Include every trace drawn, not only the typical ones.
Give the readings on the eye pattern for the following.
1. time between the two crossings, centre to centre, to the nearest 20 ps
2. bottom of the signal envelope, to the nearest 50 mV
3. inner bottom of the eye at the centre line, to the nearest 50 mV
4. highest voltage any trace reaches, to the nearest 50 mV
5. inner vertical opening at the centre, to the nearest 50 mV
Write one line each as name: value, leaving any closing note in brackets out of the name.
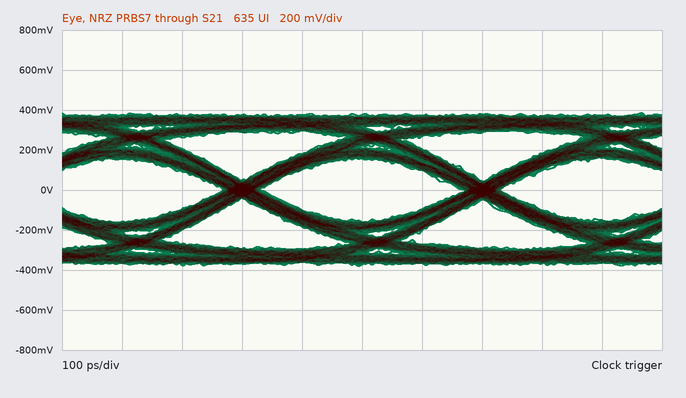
time between the two crossings, centre to centre, to the nearest 20 ps: 400 ps
bottom of the signal envelope, to the nearest 50 mV: -400 mV
inner bottom of the eye at the centre line, to the nearest 50 mV: -150 mV
highest voltage any trace reaches, to the nearest 50 mV: 400 mV
inner vertical opening at the centre, to the nearest 50 mV: 300 mV
